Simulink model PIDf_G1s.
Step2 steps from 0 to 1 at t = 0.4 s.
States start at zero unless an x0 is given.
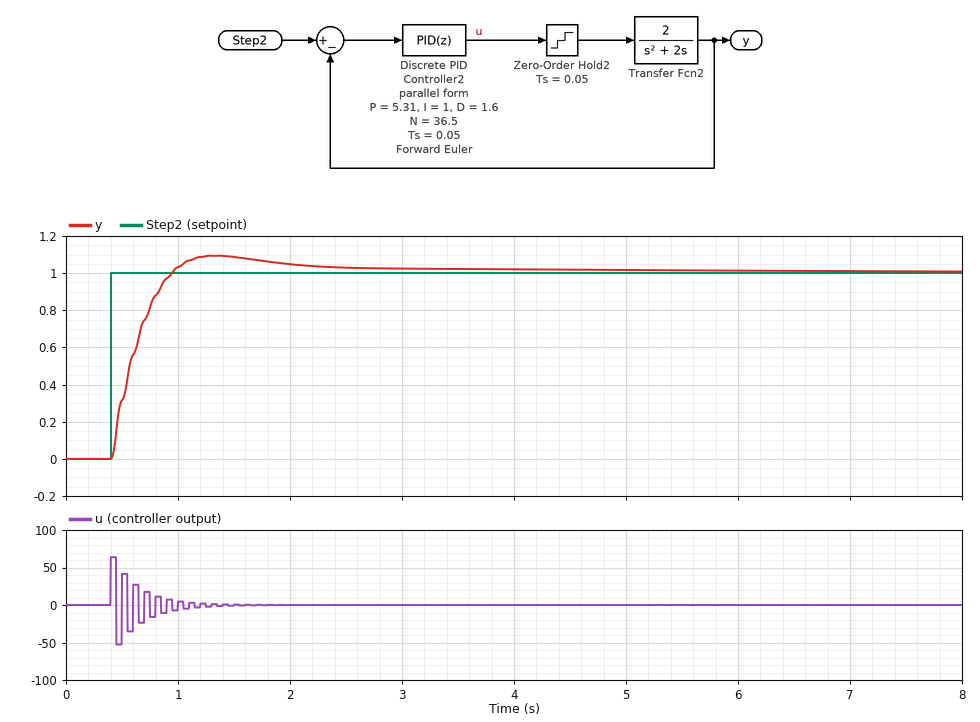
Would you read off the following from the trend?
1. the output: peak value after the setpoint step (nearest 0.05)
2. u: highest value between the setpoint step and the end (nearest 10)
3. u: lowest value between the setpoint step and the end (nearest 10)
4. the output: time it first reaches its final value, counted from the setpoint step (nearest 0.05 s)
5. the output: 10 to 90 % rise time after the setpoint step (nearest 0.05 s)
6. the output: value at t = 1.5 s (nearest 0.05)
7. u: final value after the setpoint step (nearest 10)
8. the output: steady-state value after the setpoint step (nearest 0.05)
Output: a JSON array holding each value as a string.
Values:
["1.10", "60", "-50", "0.55 s", "0.40 s", "1.10", "0", "1.00"]
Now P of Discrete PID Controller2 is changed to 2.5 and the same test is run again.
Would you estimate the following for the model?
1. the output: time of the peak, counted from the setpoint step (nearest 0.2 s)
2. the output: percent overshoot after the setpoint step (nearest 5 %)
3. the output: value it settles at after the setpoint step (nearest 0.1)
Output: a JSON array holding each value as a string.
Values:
["2.6 s", "10 %", "1.0"]
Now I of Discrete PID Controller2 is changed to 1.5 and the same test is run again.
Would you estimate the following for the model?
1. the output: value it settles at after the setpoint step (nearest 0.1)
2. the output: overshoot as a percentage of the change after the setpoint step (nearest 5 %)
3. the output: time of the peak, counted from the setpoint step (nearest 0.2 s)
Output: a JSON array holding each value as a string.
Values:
["1.0", "10 %", "1.0 s"]
